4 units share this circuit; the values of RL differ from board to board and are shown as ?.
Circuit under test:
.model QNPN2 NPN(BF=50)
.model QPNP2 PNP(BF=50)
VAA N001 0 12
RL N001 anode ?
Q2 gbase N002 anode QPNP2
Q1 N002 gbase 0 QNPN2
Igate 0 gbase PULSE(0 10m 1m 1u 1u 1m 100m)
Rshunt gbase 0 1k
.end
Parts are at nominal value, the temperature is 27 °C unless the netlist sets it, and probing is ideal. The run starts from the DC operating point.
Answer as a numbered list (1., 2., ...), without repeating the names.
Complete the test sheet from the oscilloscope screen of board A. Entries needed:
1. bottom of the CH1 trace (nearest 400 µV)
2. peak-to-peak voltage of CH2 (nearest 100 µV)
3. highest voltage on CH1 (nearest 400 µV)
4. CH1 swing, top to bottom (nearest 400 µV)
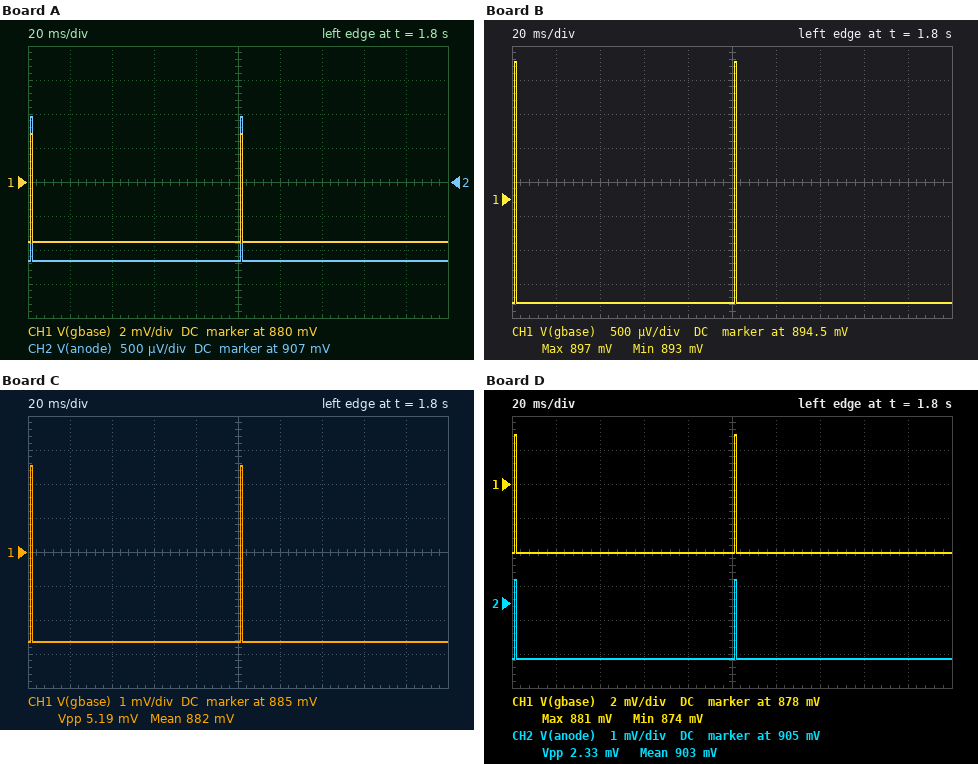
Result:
1. 876.4 mV
2. 2.1 mV
3. 882.8 mV
4. 6.4 mV
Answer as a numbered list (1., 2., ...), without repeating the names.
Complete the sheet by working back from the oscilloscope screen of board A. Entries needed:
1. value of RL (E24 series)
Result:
1. 300 Ω
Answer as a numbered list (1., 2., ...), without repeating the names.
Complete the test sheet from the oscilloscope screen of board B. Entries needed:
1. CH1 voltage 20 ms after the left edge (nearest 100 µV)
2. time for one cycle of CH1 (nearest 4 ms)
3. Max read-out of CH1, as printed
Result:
1. 893.0 mV
2. 100 ms
3. 897 mV
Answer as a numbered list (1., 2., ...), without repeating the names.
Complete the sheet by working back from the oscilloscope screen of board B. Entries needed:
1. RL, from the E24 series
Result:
1. 160 Ω
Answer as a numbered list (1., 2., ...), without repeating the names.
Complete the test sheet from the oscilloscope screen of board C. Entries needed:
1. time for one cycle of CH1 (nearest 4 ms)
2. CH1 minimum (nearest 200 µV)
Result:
1. 100 ms
2. 882.4 mV
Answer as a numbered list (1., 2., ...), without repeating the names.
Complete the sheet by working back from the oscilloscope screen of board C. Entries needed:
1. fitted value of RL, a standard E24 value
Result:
1. 240 Ω
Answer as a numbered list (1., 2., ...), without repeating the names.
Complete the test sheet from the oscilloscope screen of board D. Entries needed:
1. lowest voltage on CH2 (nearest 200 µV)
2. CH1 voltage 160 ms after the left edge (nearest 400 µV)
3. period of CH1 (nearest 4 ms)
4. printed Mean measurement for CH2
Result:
1. 903.4 mV
2. 874.0 mV
3. 100 ms
4. 903 mV
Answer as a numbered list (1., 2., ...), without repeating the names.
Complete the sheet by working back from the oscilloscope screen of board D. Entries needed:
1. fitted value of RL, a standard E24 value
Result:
1. 330 Ω
